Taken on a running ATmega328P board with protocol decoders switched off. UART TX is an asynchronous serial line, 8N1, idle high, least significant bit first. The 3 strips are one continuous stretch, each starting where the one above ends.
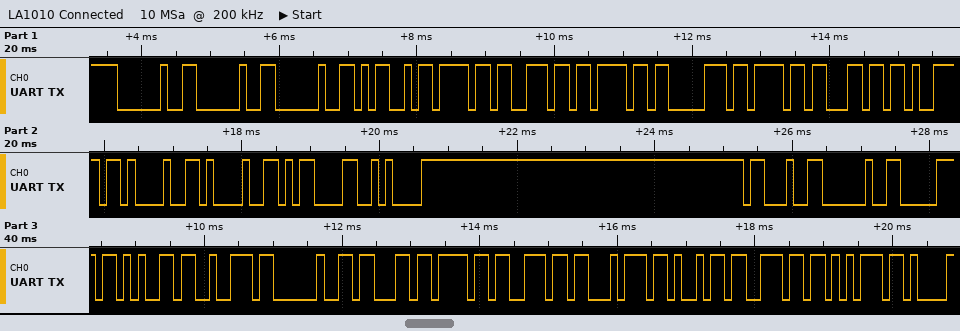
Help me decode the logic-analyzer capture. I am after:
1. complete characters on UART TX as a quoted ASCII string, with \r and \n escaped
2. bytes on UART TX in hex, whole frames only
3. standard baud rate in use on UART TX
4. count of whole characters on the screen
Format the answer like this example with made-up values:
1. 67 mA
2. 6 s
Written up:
1. "   Monopoly!!\r\n# per continu"
2. 20 20 20 4D 6F 6E 6F 70 6F 6C 79 21 21 0D 0A 23 20 70 65 72 20 63 6F 6E 74 69 6E 75
3. 9600 baud
4. 28
